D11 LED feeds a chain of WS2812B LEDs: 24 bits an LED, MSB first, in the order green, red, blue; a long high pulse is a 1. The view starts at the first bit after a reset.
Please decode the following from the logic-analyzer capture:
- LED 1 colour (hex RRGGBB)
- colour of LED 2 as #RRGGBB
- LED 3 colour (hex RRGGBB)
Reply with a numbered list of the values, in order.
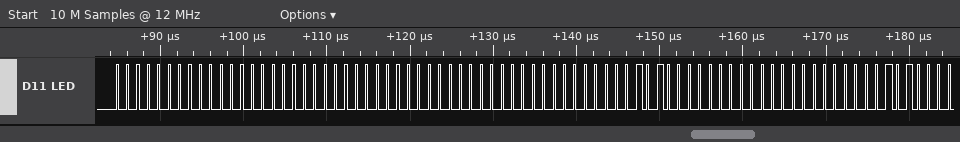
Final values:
1. #000000
2. #000000
3. #002800
